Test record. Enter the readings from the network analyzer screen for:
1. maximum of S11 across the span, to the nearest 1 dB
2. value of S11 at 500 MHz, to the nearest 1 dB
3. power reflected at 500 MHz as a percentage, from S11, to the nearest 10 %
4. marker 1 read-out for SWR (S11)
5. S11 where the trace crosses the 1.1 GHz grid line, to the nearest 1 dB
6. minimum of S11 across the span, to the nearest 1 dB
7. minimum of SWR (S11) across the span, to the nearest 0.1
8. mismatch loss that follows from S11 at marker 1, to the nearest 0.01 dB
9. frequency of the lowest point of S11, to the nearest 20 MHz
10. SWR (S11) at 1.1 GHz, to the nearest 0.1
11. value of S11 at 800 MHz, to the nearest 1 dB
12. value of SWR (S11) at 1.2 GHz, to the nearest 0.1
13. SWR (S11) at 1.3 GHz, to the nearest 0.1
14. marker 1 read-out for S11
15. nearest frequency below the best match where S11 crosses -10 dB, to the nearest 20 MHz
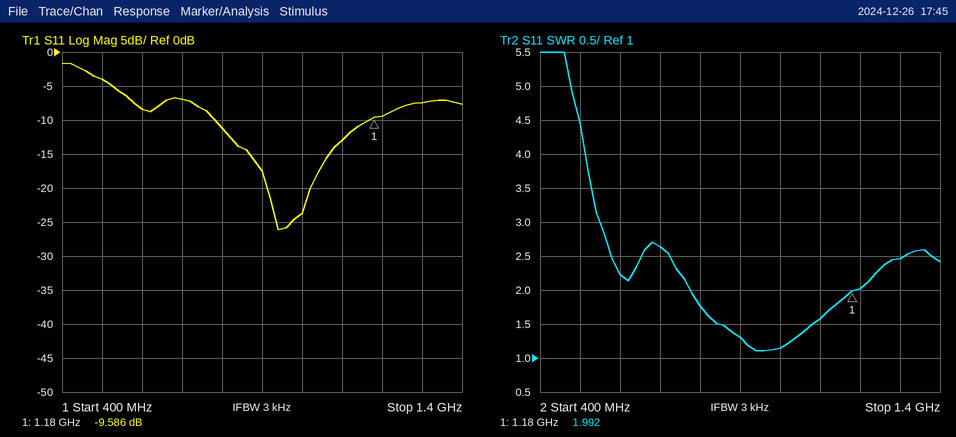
-2 dB
-4 dB
40 %
1.992
-13 dB
-26 dB
1.1
0.51 dB
940 MHz
1.6
-11 dB
2.0
2.5
-9.586 dB
780 MHz
